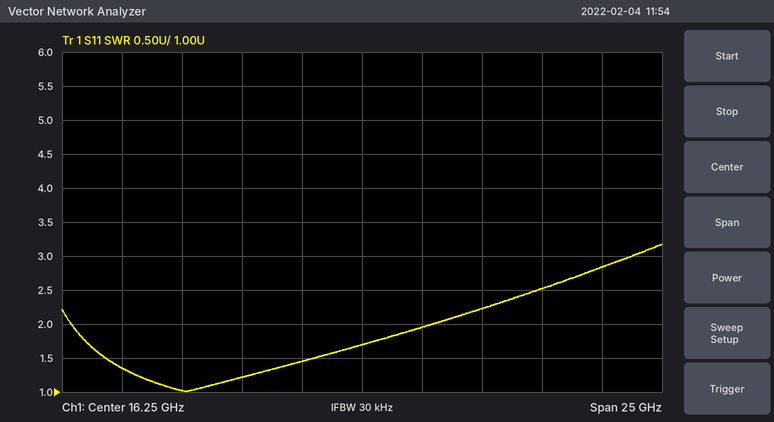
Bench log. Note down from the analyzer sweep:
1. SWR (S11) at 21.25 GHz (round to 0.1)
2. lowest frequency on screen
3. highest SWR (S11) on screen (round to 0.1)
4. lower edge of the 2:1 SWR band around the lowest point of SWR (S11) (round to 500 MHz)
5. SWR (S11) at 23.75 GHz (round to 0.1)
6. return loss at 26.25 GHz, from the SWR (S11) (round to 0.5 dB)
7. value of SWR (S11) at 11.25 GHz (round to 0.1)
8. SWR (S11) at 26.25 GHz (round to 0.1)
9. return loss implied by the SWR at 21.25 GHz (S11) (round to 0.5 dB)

2.2
3.75 GHz
3.2
4.0 GHz
2.5
6.5 dB
1.2
2.8
8.5 dB
